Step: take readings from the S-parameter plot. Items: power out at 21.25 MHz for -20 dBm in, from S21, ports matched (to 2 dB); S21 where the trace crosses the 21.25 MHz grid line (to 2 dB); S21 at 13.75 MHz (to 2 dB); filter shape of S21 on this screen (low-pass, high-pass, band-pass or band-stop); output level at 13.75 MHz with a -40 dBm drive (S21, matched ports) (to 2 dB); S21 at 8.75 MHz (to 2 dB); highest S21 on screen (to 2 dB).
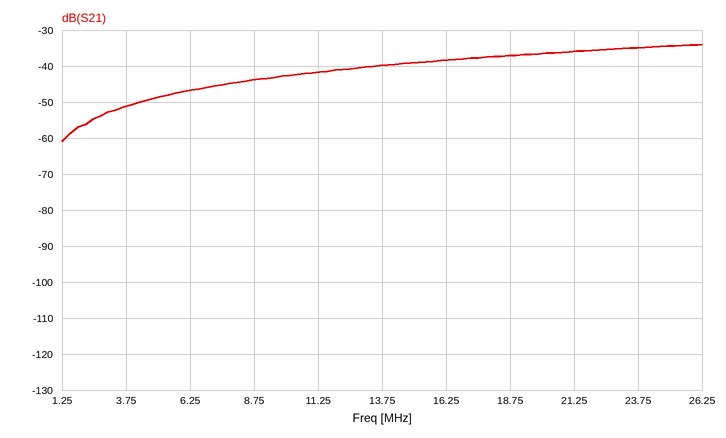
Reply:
-56 dBm
-36 dB
-40 dB
high-pass
-80 dBm
-44 dB
-34 dB
